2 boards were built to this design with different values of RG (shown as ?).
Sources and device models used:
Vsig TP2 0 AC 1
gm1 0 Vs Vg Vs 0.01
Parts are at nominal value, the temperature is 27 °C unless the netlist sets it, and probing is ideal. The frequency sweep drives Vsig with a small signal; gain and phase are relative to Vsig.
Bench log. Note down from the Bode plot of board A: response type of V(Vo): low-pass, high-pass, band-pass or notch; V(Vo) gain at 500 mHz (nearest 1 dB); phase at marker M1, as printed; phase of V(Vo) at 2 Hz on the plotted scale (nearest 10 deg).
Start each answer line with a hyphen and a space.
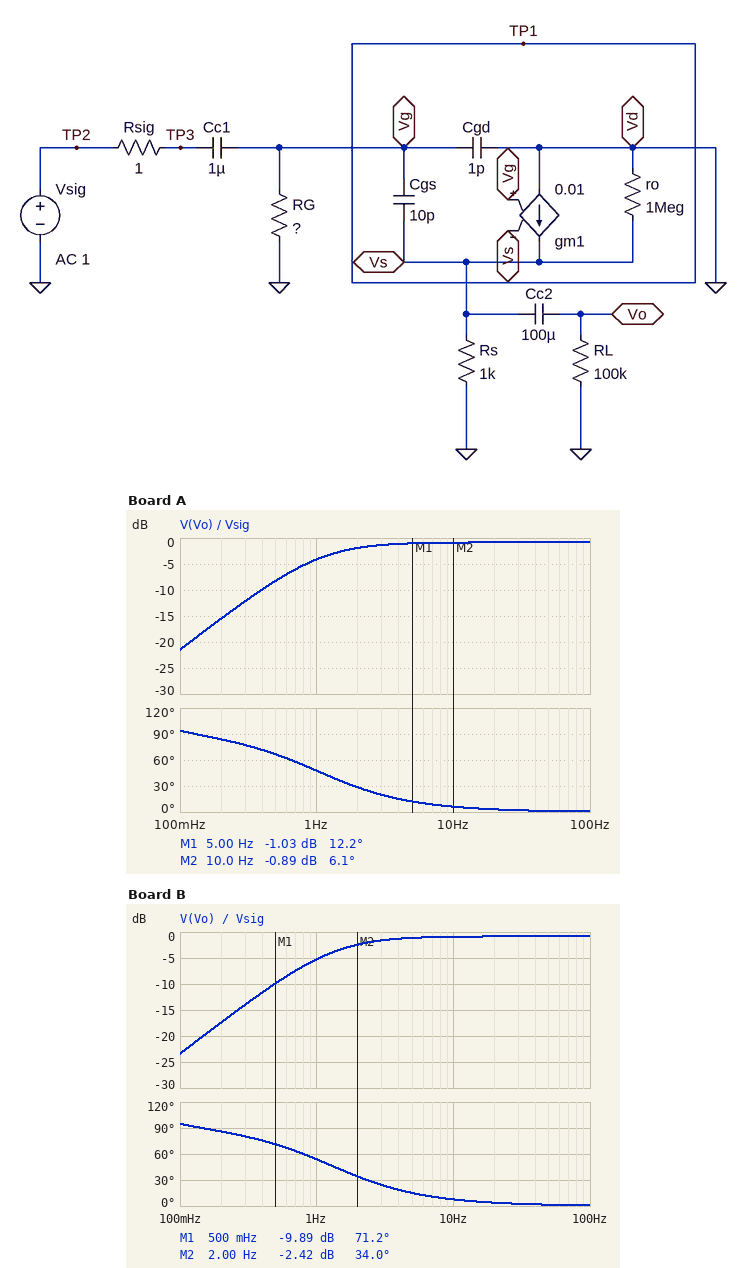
- high-pass
- -8 dB
- 12.2 deg
- 30 deg
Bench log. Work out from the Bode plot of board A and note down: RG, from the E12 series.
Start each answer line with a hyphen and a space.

- 150 kΩ
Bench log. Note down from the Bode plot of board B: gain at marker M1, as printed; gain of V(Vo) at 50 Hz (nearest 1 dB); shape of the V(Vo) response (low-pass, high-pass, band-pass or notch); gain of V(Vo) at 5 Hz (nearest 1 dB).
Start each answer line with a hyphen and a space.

- -9.89 dB
- -1 dB
- high-pass
- -1 dB
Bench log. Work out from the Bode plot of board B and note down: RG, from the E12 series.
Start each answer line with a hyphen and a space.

- 120 kΩ
